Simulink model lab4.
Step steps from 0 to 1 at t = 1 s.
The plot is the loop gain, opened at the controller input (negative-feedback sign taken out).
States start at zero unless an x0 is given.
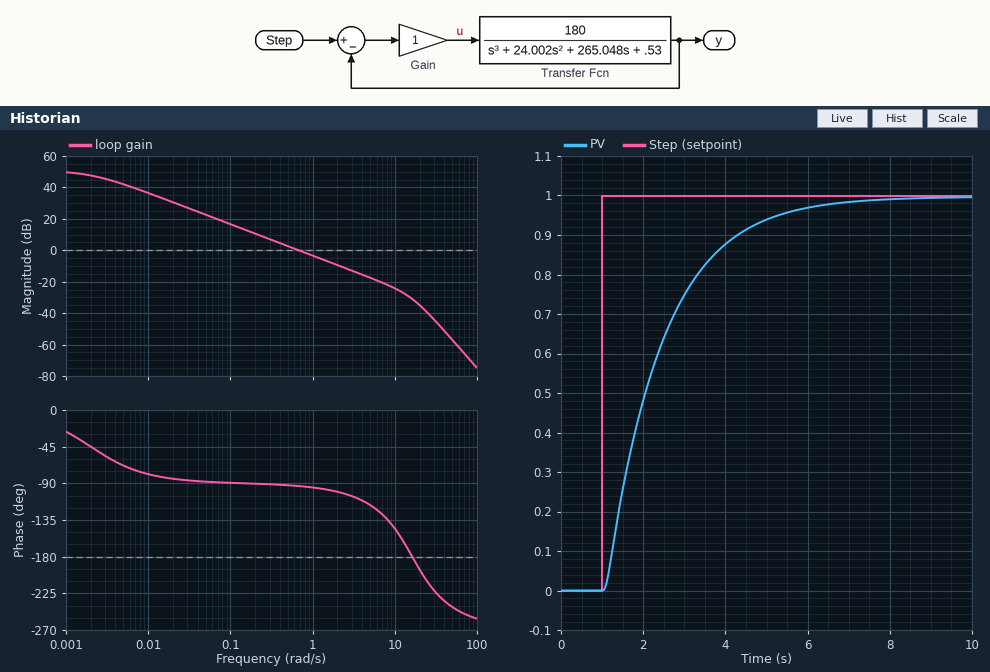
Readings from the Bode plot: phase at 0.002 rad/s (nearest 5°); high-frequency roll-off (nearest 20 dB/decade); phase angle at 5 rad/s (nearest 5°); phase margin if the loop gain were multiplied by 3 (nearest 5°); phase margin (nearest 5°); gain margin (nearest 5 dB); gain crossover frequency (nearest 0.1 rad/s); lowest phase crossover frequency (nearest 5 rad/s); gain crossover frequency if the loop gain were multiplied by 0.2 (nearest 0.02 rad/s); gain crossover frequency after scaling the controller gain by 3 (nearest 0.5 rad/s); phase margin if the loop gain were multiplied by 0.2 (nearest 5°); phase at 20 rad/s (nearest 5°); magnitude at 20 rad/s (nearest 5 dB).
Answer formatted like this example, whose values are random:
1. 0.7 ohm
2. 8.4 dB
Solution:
1. -45°
2. -60 dB/decade
3. -115°
4. 80°
5. 85°
6. 30 dB
7. 0.7 rad/s
8. 15 rad/s
9. 0.14 rad/s
10. 2.0 rad/s
11. 90°
12. -195°
13. -35 dB
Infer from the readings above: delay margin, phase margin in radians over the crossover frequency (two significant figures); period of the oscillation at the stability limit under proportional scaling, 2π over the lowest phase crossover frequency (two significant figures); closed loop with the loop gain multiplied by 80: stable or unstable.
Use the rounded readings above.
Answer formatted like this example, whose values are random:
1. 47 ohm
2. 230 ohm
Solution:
1. 2.1 s
2. 0.42 s
3. unstable
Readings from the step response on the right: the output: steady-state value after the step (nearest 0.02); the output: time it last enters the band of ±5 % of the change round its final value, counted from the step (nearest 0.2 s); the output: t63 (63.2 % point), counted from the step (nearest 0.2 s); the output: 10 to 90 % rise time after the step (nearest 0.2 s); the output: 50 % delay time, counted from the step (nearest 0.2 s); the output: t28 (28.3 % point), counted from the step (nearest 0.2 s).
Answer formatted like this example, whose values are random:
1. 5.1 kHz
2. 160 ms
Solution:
1. 1.00
2. 4.2 s
3. 1.4 s
4. 3.0 s
5. 1.0 s
6. 0.6 s
